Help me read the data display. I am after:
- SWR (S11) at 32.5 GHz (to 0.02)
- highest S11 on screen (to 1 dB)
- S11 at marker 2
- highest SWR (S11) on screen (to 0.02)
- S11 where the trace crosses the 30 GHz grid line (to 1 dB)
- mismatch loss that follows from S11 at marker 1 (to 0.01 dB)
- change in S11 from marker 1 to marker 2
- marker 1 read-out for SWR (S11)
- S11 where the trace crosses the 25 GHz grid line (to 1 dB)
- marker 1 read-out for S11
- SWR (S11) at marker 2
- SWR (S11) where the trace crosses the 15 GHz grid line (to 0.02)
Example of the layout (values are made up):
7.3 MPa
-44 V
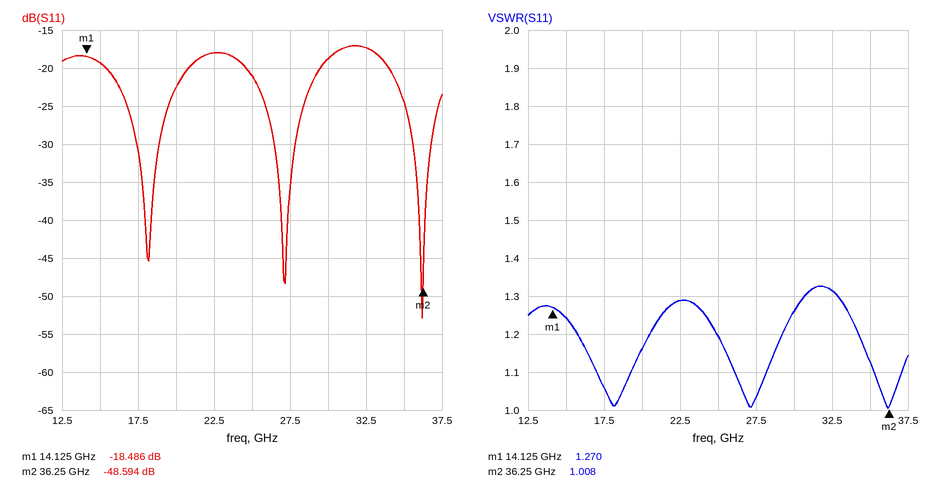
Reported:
1.32
-17 dB
-48.594 dB
1.32
-19 dB
0.06 dB
-30.108 dB
1.270
-21 dB
-18.486 dB
1.008
1.24
